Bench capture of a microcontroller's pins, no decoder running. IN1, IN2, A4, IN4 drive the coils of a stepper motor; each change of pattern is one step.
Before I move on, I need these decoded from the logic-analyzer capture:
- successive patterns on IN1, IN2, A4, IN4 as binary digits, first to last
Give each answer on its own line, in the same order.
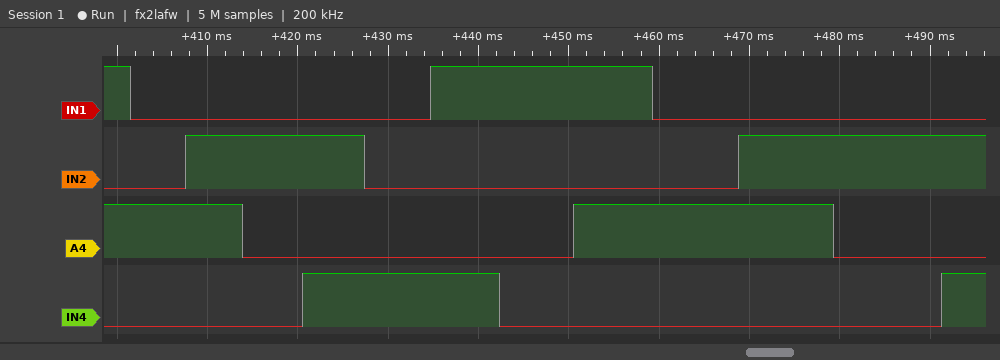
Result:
1010 0010 0110 0100 0101 0001 1001 1000 1010 0010 0110 0100 0101
